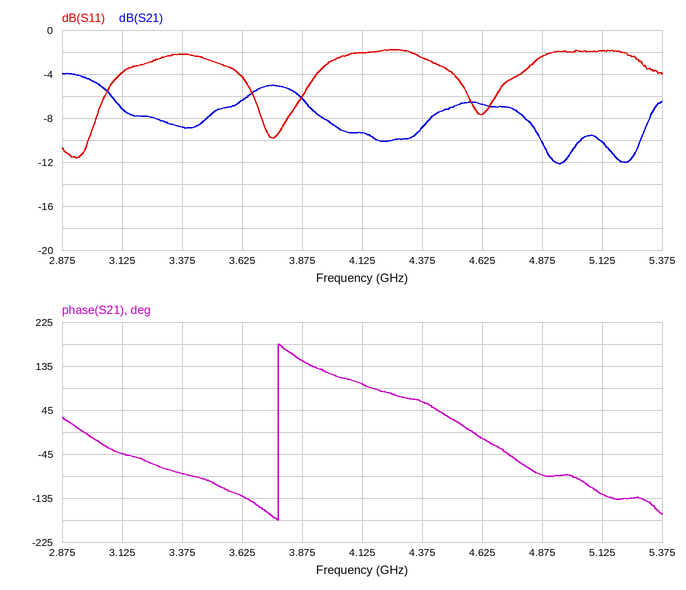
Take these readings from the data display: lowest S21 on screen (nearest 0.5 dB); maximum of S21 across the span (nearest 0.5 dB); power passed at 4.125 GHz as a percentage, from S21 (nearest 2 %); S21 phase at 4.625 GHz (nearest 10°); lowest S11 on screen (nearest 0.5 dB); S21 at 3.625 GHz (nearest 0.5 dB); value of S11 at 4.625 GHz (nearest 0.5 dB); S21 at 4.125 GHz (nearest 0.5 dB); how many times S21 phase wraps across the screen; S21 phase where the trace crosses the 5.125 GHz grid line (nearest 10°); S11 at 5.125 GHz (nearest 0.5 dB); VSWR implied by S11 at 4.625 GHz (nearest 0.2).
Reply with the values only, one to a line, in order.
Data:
-12.0 dB
-4.0 dB
12 %
-10°
-11.5 dB
-6.5 dB
-7.5 dB
-9.5 dB
1
-130°
-2.0 dB
2.4
